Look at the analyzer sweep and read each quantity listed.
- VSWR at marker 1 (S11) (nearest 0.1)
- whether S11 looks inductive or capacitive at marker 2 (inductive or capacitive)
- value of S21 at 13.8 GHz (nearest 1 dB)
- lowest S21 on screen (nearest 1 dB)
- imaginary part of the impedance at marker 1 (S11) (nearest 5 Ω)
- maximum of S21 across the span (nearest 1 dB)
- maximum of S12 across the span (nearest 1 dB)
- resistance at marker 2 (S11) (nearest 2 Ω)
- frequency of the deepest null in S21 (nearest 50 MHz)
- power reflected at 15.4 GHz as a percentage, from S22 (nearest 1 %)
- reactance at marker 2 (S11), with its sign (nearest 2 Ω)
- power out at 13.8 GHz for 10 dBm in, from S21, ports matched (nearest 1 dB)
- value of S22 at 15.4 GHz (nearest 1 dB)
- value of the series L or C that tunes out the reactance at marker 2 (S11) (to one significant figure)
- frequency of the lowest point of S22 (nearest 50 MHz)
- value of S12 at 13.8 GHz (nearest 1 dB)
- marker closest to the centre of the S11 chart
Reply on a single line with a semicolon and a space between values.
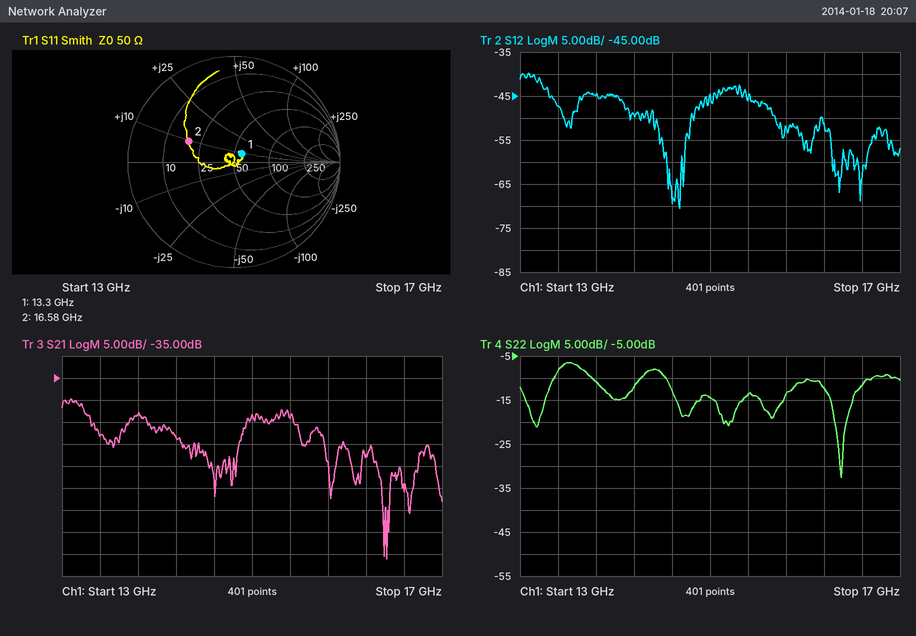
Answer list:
1.2; inductive; -43 dB; -76 dB; +10 Ω; -40 dB; -40 dB; 18 Ω; 16.40 GHz; 4 %; +10 Ω; -33 dBm; -14 dB; 1 pF; 16.40 GHz; -45 dB; marker 1
